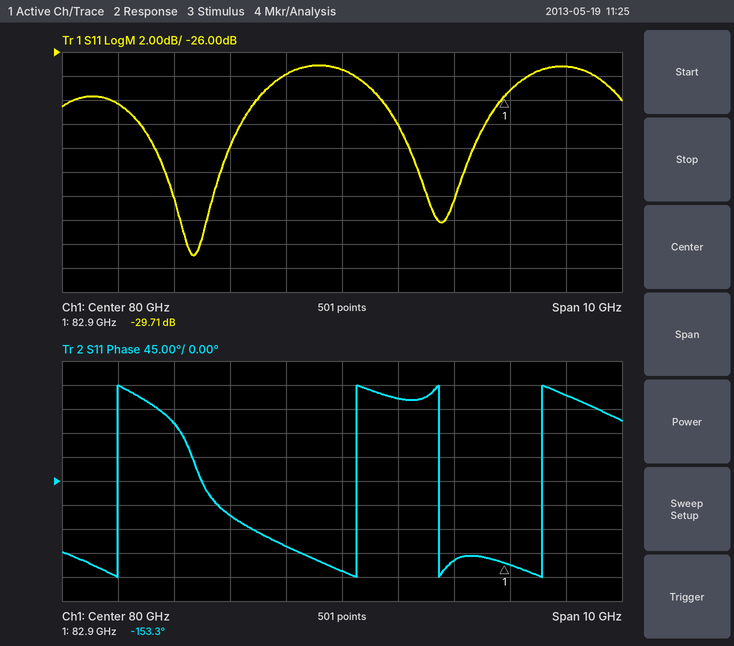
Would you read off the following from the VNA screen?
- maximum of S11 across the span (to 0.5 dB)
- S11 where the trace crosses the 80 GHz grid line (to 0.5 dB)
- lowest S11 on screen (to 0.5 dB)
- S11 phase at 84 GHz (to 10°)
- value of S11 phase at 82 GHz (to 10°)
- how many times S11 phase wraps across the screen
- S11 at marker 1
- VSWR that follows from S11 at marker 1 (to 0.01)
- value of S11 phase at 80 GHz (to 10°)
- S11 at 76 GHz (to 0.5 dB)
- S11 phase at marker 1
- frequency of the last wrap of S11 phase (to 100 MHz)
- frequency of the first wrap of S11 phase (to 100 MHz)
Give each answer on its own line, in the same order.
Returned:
-27.0 dB
-27.5 dB
-43.0 dB
160°
-150°
4
-29.71 dB
1.07
-170°
-30.5 dB
-153.3°
83.6 GHz
76.0 GHz
